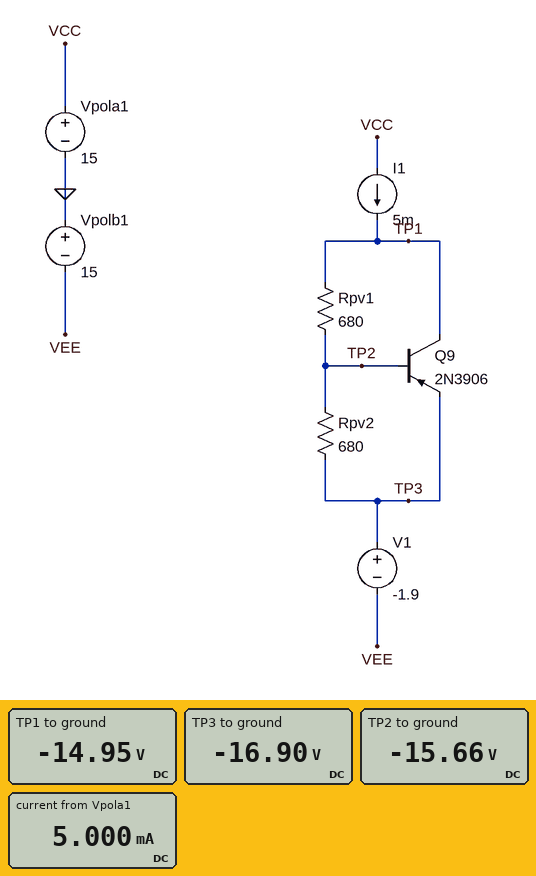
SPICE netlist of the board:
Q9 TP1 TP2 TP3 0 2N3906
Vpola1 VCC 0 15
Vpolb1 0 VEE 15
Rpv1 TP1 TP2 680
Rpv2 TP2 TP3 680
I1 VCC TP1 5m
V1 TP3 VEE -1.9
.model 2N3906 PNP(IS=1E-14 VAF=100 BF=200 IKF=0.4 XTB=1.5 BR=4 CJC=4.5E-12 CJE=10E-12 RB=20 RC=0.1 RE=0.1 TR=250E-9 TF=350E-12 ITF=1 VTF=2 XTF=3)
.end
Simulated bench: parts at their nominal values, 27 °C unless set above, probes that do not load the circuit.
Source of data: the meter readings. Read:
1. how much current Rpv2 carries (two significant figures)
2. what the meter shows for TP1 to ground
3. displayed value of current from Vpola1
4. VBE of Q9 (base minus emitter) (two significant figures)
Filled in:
1.8 mA
-14.95 V
5.000 mA
1.2 V
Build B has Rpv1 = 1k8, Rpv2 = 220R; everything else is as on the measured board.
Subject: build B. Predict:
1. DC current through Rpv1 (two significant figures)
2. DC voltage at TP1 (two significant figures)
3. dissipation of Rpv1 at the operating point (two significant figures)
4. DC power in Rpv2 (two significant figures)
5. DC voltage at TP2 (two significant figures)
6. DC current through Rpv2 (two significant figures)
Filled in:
390 µA
-16 V
280 µW
380 µW
-17 V
1.3 mA
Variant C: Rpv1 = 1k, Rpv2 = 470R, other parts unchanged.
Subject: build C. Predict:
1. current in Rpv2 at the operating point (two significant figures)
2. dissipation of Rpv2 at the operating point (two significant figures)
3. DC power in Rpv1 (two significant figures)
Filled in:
1.6 mA
1.2 mW
500 µW
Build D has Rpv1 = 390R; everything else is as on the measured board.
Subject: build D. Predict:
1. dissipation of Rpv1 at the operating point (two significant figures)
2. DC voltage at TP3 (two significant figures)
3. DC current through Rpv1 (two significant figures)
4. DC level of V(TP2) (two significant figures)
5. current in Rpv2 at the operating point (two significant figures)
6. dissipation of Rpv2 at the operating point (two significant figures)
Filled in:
1.2 mW
-17 V
1.8 mA
-15 V
2.4 mA
4.0 mW
